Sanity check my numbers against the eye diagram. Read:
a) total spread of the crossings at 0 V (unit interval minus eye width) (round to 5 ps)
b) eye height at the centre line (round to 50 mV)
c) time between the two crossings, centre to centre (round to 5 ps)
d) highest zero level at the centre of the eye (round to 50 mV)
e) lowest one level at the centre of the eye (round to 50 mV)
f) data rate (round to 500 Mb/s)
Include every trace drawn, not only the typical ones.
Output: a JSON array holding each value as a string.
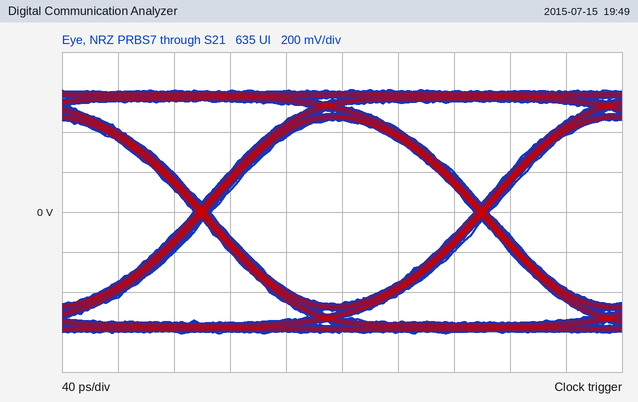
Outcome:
["10 ps", "900 mV", "200 ps", "-450 mV", "450 mV", "5.0 Gb/s"]
